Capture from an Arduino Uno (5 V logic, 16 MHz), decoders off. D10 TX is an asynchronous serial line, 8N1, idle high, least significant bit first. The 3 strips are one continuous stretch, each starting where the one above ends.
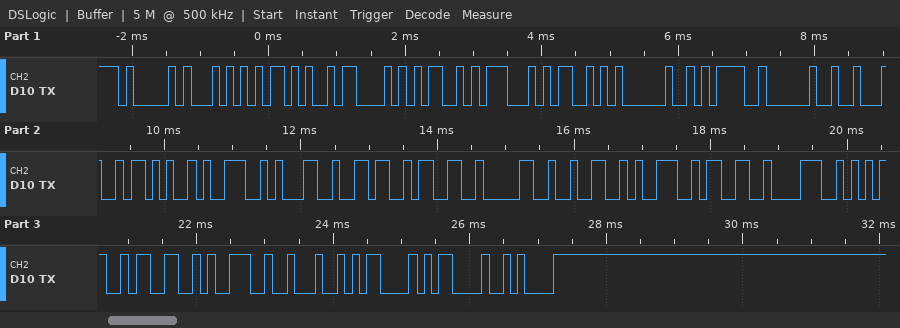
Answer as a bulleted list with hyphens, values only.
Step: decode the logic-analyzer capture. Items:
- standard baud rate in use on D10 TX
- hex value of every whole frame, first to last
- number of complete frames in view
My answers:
- 9600 baud
- 0x41 0x54 0x2B 0x43 0x4D 0x47 0x53 0x20 0x3D 0x20 0x22 0x2B 0x39 0x31 0x36 0x33 0x30 0x32 0x39 0x33 0x38 0x35 0x33 0x39 0x22 0x0D 0x0D 0x0A
- 28
